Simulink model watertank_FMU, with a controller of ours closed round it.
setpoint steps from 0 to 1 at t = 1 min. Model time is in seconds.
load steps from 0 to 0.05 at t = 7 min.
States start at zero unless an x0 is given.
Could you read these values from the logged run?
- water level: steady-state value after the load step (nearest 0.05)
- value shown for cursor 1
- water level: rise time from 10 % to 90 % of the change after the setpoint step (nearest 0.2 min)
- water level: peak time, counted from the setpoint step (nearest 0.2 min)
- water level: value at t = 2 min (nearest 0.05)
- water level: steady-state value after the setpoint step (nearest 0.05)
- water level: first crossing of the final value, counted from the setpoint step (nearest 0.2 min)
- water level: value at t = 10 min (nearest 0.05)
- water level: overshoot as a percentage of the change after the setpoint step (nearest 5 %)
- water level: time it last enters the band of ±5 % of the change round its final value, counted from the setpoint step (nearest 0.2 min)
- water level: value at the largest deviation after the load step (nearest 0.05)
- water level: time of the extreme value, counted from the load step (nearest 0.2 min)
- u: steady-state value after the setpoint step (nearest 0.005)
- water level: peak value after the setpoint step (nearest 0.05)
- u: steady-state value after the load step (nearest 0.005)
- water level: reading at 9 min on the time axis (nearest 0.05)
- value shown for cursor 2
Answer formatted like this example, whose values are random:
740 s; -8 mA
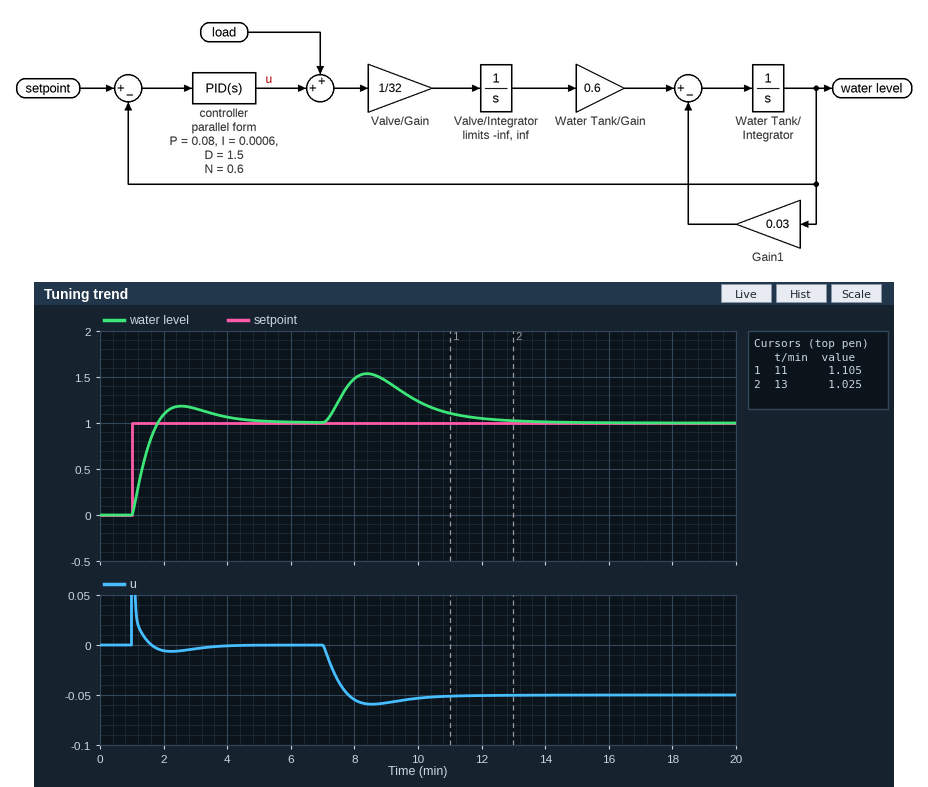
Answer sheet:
1.00; 1.105; 0.6 min; 1.6 min; 1.10; 1.00; 0.8 min; 1.25; 20 %; 3.2 min; 1.55; 1.4 min; 0.000; 1.20; -0.050; 1.45; 1.025
